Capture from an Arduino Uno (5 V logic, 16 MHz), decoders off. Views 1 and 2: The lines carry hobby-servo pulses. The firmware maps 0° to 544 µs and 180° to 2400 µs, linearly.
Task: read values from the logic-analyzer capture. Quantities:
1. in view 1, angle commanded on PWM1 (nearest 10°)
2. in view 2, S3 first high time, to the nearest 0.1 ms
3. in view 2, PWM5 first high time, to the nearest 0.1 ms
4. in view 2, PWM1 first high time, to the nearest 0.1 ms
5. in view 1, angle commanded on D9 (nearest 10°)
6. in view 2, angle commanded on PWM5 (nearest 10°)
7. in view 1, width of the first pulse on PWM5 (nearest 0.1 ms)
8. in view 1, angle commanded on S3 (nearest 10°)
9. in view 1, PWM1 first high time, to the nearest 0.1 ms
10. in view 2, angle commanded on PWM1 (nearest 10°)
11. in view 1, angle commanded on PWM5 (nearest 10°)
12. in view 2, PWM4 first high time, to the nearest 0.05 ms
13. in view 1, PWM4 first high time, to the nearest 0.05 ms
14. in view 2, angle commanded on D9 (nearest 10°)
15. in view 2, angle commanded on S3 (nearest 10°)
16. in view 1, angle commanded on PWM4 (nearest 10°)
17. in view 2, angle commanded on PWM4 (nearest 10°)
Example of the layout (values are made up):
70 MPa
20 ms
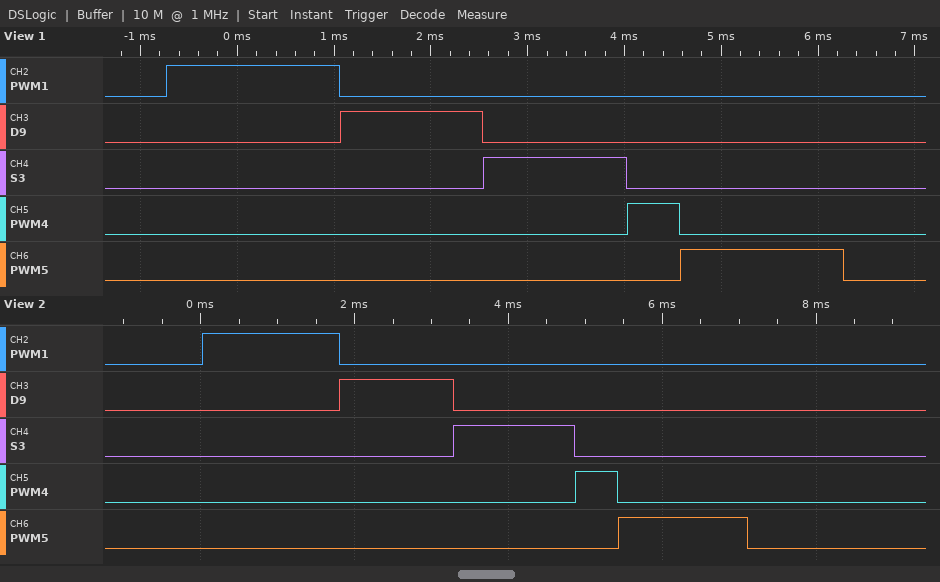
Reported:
120°
1.6 ms
1.7 ms
1.8 ms
90°
110°
1.7 ms
90°
1.8 ms
120°
110°
0.55 ms
0.55 ms
90°
100°
0°
0°
